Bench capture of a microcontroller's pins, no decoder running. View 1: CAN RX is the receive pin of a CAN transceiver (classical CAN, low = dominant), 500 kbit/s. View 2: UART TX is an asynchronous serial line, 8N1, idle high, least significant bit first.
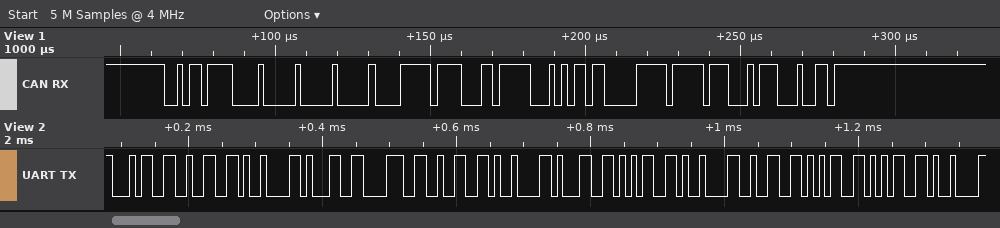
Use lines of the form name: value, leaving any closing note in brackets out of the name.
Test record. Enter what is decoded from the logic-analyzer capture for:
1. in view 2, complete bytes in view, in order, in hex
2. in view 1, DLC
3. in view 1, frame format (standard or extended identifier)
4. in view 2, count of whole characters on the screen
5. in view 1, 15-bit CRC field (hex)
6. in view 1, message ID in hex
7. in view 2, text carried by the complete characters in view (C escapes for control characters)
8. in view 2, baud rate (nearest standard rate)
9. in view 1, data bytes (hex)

in view 2, complete bytes in view, in order, in hex: 0x34 0x32 0x09 0x31 0x38 0x32 0x09 0x31 0x35 0x09 0x32 0x35 0x35 0x09
in view 1, DLC: 8
in view 1, frame format: standard
in view 2, count of whole characters on the screen: 14
in view 1, 15-bit CRC field: 0x0B89
in view 1, message ID in hex: 0x2DE
in view 2, text carried by the complete characters in view: "42\t182\t15\t255\t"
in view 2, baud rate: 115200 baud
in view 1, data bytes: 00 00 FF 8D F2 B6 0F FF
